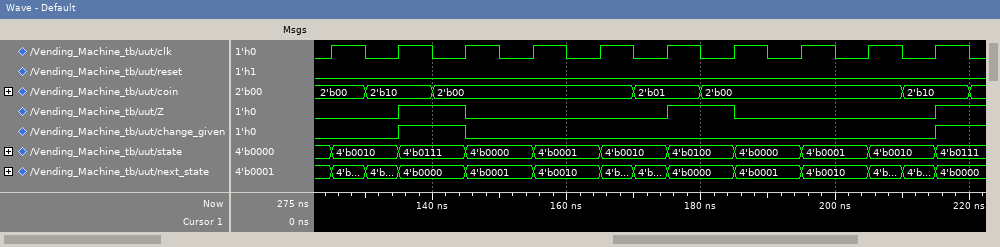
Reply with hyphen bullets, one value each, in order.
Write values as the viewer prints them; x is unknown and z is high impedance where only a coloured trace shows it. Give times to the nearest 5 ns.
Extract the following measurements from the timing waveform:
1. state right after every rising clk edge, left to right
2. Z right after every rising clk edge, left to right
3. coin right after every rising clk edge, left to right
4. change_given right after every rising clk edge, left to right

- 4'b0010, 4'b0111, 4'b0000, 4'b0001, 4'b0010, 4'b0100, 4'b0000, 4'b0001, 4'b0010, 4'b0111
- 0 1 0 0 0 1 0 0 0 1
- 2'b00, 2'b10, 2'b00, 2'b00, 2'b00, 2'b01, 2'b00, 2'b00, 2'b00, 2'b10
- 0 1 0 0 0 0 0 0 0 1
